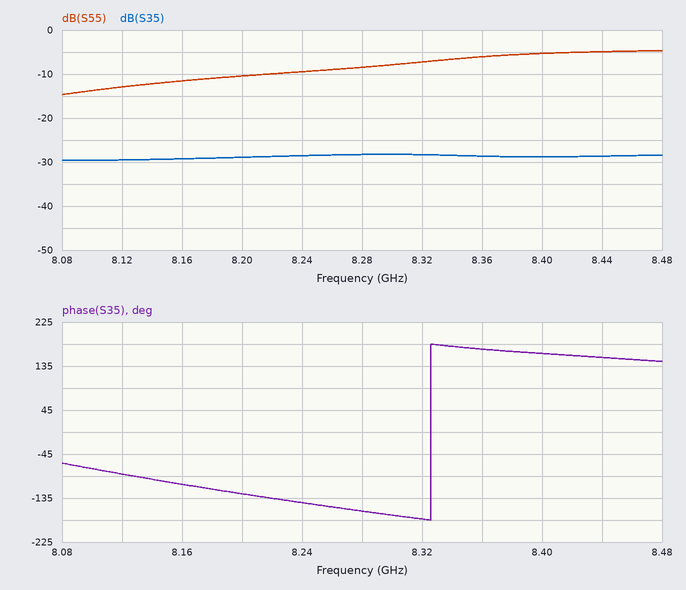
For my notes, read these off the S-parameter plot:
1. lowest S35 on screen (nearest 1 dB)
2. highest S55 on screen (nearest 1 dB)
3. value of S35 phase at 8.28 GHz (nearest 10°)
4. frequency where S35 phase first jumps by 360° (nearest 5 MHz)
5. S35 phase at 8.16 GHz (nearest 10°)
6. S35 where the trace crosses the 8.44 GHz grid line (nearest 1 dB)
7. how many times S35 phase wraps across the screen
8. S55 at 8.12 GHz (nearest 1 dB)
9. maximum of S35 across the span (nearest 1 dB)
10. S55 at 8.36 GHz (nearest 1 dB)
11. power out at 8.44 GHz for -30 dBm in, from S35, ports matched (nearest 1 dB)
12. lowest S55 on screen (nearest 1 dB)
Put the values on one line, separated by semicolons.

-30 dB; -5 dB; -160°; 8.325 GHz; -110°; -29 dB; 1; -13 dB; -28 dB; -6 dB; -59 dBm; -15 dB
